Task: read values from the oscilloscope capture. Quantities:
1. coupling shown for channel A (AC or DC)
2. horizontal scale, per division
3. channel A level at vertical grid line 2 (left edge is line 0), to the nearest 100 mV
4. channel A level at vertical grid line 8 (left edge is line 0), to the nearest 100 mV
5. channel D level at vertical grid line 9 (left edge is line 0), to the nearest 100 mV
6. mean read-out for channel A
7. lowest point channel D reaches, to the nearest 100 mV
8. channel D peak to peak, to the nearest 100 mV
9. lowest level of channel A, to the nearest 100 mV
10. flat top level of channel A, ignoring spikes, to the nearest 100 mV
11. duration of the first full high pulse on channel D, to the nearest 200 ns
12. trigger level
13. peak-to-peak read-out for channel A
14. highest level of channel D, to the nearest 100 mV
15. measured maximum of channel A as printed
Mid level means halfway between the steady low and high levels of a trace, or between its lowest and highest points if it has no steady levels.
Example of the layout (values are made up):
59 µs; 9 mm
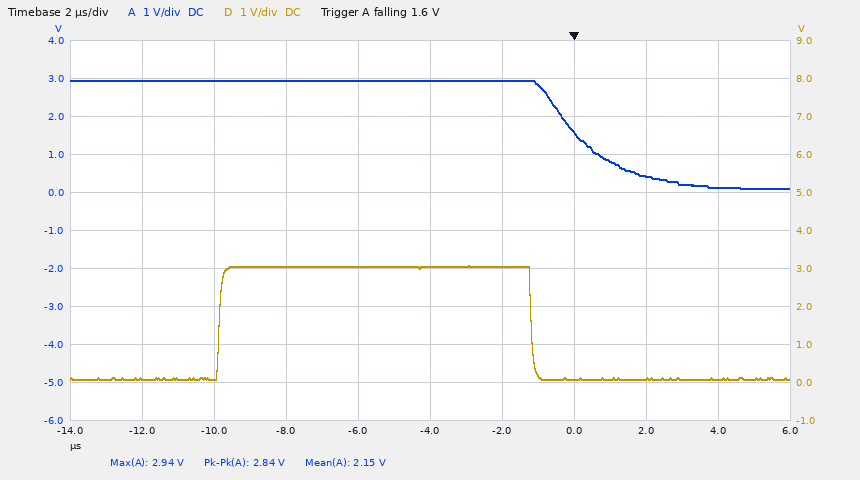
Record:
DC; 2 µs; 2.9 V; 400 mV; 100 mV; 2.15 V; 100 mV; 3.0 V; 100 mV; 2.9 V; 8.6 µs; 1.6 V; 2.84 V; 3.1 V; 2.94 V
